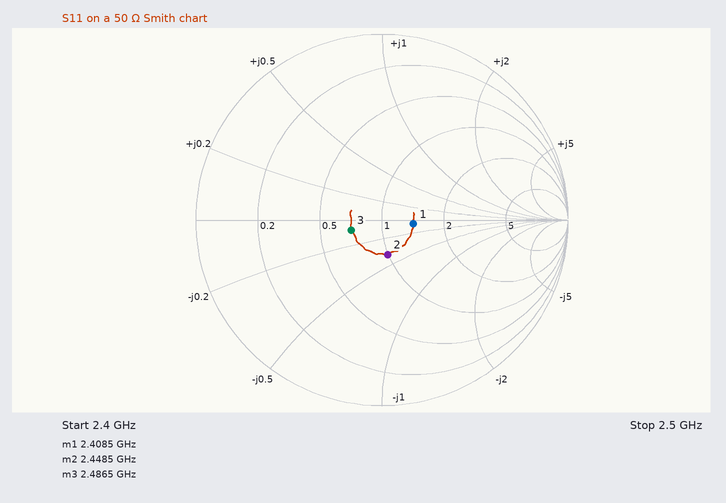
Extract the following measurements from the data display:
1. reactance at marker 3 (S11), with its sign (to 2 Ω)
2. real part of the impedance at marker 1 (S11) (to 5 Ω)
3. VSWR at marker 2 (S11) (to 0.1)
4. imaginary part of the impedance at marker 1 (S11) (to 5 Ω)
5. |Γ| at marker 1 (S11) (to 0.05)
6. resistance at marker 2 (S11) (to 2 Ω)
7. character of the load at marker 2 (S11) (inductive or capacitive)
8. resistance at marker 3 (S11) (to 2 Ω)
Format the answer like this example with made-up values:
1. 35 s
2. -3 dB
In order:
1. -4 Ω
2. 70 Ω
3. 1.5
4. -5 Ω
5. 0.15
6. 50 Ω
7. capacitive
8. 36 Ω
